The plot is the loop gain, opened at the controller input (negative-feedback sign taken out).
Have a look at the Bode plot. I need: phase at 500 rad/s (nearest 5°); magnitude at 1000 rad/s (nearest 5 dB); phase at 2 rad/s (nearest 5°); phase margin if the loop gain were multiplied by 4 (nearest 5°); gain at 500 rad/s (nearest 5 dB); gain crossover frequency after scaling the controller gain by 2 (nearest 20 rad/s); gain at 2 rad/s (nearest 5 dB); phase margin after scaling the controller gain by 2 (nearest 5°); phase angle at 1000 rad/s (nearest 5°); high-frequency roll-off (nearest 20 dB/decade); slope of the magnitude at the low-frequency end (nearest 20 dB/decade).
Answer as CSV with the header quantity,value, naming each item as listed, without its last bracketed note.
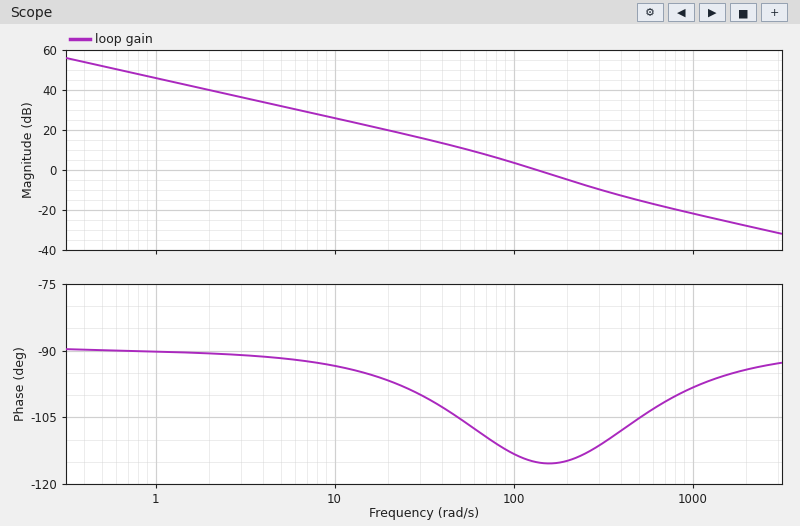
quantity,value
phase at 500 rad/s,-105°
magnitude at 1000 rad/s,-20 dB
phase at 2 rad/s,-90°
phase margin if the loop gain were multiplied by 4,70°
gain at 500 rad/s,-15 dB
gain crossover frequency after scaling the controller gain by 2,220 rad/s
gain at 2 rad/s,40 dB
phase margin after scaling the controller gain by 2,65°
phase angle at 1000 rad/s,-100°
high-frequency roll-off,-20 dB/decade
slope of the magnitude at the low-frequency end,-20 dB/decade
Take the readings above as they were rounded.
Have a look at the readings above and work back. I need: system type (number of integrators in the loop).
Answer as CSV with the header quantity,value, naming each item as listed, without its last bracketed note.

quantity,value
system type,1
